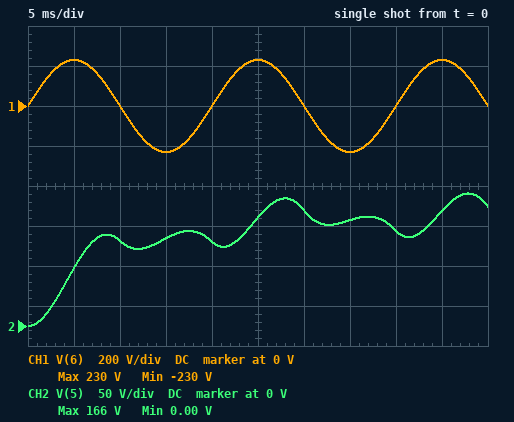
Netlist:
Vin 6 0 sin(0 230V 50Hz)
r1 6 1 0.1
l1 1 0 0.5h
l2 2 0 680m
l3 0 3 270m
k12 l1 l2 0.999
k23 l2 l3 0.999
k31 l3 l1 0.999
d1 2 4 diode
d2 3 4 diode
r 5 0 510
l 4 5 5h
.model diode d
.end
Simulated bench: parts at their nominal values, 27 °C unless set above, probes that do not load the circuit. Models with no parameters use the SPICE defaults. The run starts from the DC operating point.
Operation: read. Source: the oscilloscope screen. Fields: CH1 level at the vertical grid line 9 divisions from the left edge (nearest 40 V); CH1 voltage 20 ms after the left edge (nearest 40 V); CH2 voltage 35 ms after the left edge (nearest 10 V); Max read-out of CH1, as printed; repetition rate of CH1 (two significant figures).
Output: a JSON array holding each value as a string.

["240 V", "0 V", "130 V", "230 V", "50 Hz"]
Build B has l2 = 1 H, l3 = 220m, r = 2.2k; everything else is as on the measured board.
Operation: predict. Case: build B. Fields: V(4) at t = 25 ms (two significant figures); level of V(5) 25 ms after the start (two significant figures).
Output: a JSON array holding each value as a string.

["320 V", "240 V"]
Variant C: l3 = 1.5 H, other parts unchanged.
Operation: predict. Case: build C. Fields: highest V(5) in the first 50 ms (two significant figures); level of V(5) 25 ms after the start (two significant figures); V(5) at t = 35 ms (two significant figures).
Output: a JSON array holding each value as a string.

["250 V", "190 V", "210 V"]
